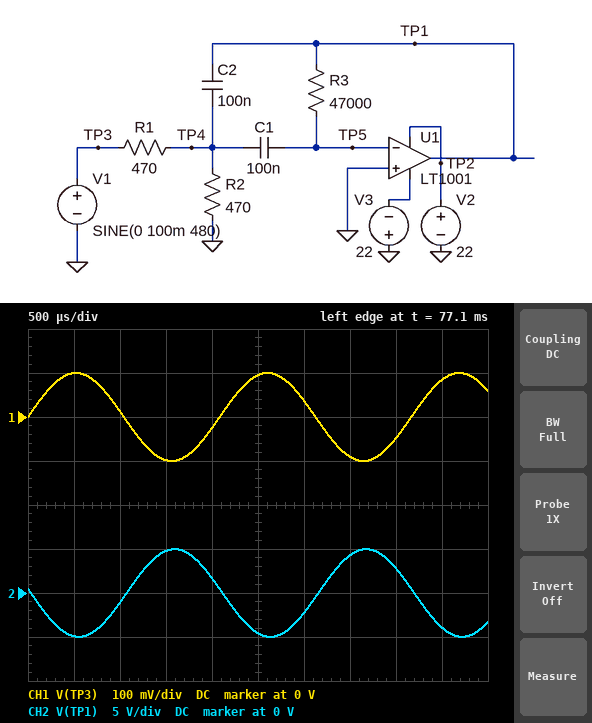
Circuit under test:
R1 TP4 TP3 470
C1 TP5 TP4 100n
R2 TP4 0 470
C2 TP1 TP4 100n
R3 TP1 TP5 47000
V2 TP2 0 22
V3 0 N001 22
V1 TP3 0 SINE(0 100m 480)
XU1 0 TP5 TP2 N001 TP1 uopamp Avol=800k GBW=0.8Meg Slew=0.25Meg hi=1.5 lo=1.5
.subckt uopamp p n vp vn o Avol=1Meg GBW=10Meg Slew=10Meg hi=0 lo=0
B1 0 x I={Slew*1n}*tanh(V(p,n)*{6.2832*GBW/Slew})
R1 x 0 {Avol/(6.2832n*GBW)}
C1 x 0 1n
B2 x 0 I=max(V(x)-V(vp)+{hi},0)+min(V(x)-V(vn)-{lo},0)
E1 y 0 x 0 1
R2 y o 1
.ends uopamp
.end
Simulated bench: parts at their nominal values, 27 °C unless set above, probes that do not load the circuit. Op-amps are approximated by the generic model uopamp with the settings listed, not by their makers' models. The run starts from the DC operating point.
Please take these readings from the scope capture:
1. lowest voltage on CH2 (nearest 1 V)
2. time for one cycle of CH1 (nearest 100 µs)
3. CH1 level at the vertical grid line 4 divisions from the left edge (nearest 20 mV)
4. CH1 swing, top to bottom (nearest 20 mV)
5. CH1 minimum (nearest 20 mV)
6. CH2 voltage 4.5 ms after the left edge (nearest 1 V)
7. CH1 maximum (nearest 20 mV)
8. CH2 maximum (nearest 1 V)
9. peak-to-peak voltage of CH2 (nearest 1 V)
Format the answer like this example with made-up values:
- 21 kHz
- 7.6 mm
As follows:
- -5 V
- 2.1 ms
- -20 mV
- 200 mV
- -100 mV
- -4 V
- 100 mV
- 5 V
- 10 V
